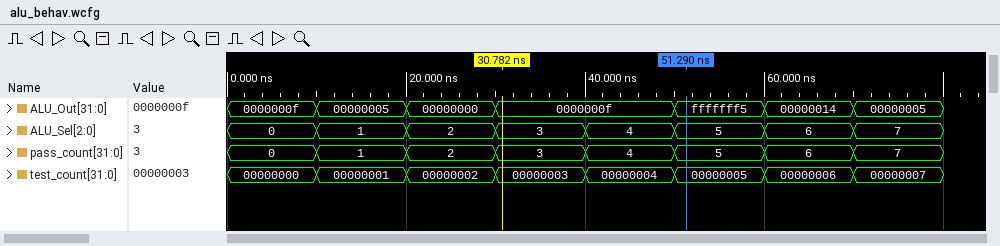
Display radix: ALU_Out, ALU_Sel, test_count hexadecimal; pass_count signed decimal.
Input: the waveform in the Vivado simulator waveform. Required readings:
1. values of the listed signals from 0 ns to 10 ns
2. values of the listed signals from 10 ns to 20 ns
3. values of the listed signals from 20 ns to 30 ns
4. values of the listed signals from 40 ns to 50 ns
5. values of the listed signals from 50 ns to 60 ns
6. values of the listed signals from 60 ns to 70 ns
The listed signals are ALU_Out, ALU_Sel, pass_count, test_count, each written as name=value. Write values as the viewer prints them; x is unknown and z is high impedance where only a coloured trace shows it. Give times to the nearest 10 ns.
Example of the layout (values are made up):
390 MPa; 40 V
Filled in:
ALU_Out=0000000f, ALU_Sel=0, pass_count=0, test_count=00000000; ALU_Out=00000005, ALU_Sel=1, pass_count=1, test_count=00000001; ALU_Out=00000000, ALU_Sel=2, pass_count=2, test_count=00000002; ALU_Out=0000000f, ALU_Sel=4, pass_count=4, test_count=00000004; ALU_Out=fffffff5, ALU_Sel=5, pass_count=5, test_count=00000005; ALU_Out=00000014, ALU_Sel=6, pass_count=6, test_count=00000006
